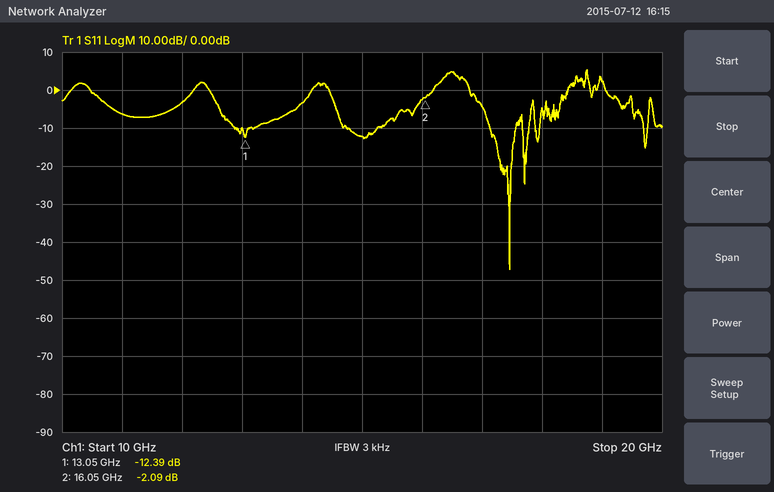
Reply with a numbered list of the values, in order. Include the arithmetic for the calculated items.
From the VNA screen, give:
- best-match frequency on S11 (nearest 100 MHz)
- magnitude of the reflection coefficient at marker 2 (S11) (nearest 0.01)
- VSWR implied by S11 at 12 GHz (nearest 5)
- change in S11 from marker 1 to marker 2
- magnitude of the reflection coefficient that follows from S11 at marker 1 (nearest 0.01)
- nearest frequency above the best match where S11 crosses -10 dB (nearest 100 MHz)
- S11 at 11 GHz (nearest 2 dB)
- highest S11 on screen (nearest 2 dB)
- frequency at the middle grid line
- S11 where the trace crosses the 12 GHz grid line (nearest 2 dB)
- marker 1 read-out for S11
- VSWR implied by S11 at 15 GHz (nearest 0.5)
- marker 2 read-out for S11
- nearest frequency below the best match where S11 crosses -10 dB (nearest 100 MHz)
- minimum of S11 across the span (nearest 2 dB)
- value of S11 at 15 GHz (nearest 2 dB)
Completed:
1. 17.5 GHz
2. 10^(-2.09/20) ≈ 0.79
3. |Γ| = 10^(-4/20) = 0.6310; VSWR = (1 + 0.6310)/(1 − 0.6310) ≈ 4.42, so 5 to the nearest 5
4. -2.09 − (-12.39) = 10.30 dB
5. 10^(-12.39/20) ≈ 0.24
6. 17.6 GHz
7. -6 dB
8. 6 dB
9. 15 GHz
10. -4 dB
11. -12.39 dB
12. |Γ| = 10^(-12/20) = 0.2512; VSWR = (1 + 0.2512)/(1 − 0.2512) ≈ 1.67, so 1.5 to the nearest 0.5
13. -2.09 dB
14. 17.1 GHz
15. -48 dB
16. -12 dB
